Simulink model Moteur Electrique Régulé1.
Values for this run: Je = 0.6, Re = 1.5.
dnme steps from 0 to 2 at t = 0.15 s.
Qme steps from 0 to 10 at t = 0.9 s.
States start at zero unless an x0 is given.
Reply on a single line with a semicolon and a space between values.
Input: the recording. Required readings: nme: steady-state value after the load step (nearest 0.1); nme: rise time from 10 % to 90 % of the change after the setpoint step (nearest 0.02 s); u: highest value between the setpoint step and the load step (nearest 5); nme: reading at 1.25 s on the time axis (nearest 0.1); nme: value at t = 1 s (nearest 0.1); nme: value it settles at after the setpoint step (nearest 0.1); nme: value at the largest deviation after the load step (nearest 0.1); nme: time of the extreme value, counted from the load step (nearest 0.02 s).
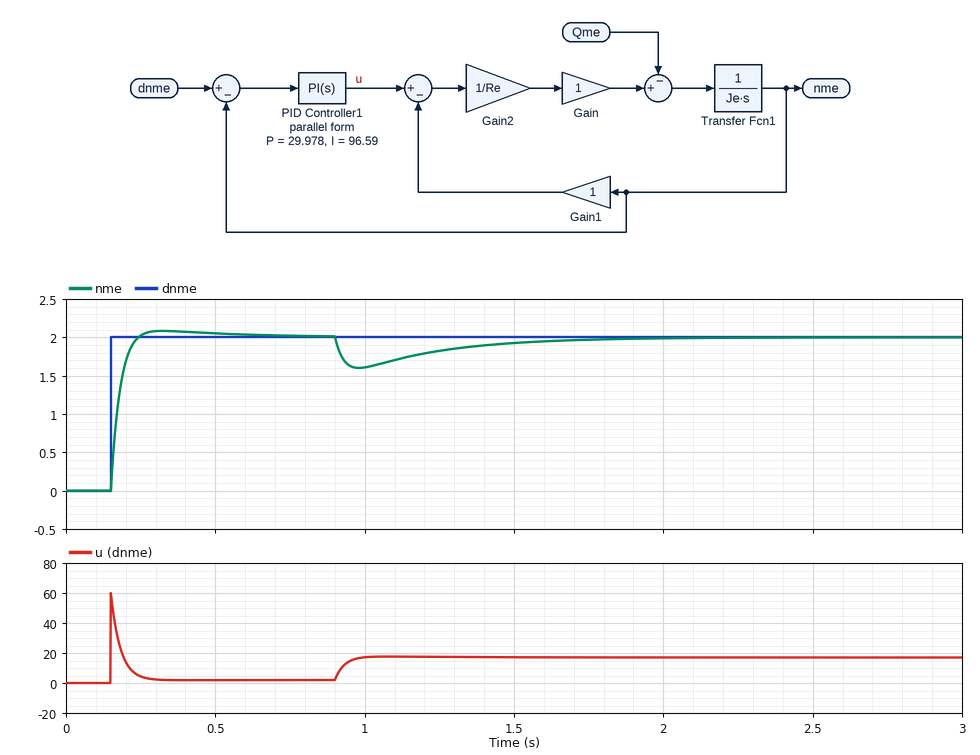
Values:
2.0; 0.06 s; 60; 1.8; 1.6; 2.0; 1.6; 0.08 s
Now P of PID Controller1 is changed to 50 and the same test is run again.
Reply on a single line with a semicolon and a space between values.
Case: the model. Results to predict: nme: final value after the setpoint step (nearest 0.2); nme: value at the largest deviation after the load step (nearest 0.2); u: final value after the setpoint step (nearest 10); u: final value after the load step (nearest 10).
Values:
2.0; 1.8; 0; 20
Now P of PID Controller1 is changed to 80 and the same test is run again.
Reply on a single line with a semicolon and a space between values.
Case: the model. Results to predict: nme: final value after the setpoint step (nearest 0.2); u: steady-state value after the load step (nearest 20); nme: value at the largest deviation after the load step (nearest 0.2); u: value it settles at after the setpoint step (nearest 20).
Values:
2.0; 20; 1.8; 0
